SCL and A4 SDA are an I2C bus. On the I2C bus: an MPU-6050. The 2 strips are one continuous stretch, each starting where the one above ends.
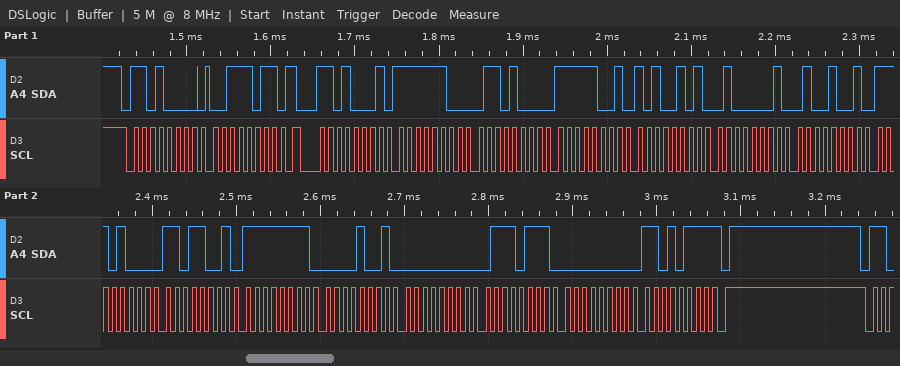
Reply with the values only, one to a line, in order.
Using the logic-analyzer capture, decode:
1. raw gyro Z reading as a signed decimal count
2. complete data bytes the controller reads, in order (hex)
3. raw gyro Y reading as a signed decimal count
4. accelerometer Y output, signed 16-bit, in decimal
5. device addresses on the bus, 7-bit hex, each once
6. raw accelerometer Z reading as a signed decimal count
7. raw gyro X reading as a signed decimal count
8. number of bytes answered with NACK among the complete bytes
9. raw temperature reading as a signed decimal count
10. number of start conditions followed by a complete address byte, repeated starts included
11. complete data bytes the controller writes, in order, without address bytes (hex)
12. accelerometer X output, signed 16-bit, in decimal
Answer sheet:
215
FC 68 F9 A5 41 49 E8 D9 FF 09 00 77 00 D7
119
-1627
0x68
16713
-247
1
-5927
2
3B
-920
